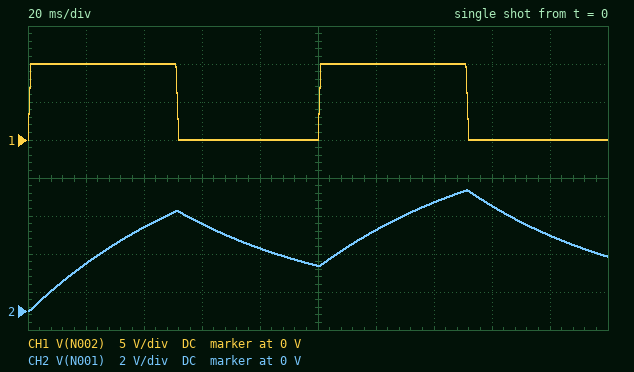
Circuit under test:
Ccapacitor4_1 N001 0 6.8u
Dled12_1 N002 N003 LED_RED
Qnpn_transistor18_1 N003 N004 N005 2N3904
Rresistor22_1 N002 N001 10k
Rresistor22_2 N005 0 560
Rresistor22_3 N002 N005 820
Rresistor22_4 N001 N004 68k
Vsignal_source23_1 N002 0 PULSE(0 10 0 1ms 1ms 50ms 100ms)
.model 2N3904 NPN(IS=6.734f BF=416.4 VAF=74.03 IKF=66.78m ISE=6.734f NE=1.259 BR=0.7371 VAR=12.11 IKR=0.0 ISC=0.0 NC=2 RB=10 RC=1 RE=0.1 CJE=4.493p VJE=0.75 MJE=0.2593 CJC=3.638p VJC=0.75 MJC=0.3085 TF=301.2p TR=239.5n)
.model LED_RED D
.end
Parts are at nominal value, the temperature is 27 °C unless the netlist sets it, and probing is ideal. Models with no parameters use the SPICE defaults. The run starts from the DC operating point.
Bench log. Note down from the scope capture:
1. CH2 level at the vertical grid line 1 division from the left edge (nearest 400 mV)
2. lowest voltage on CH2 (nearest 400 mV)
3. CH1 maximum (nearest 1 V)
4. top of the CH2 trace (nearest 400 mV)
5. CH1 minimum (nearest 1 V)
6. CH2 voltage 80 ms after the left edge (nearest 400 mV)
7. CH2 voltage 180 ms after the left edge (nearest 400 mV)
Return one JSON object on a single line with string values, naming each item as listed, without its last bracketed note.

{"CH2 level at the vertical grid line 1 division from the left edge": "2.4 V", "lowest voltage on CH2": "0 V", "CH1 maximum": "10 V", "top of the CH2 trace": "6.4 V", "CH1 minimum": "0 V", "CH2 voltage 80 ms after the left edge": "3.2 V", "CH2 voltage 180 ms after the left edge": "4.0 V"}
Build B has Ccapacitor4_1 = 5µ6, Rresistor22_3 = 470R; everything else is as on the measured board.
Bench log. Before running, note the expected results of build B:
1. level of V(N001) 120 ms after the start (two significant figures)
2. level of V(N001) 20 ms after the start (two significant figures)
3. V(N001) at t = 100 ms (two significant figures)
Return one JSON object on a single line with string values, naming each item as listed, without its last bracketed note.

{"level of V(N001) 120 ms after the start": "4.5 V", "level of V(N001) 20 ms after the start": "2.9 V", "V(N001) at t = 100 ms": "2.3 V"}
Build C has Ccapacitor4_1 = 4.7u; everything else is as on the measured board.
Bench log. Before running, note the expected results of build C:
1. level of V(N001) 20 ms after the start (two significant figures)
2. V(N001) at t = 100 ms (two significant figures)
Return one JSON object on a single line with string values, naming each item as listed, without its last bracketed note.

{"level of V(N001) 20 ms after the start": "3.4 V", "V(N001) at t = 100 ms": "2.1 V"}
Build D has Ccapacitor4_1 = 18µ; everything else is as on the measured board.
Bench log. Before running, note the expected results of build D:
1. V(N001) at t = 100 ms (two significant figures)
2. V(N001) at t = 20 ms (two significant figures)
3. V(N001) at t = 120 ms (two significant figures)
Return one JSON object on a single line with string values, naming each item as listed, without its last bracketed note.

{"V(N001) at t = 100 ms": "1.8 V", "V(N001) at t = 20 ms": "1.0 V", "V(N001) at t = 120 ms": "2.7 V"}
